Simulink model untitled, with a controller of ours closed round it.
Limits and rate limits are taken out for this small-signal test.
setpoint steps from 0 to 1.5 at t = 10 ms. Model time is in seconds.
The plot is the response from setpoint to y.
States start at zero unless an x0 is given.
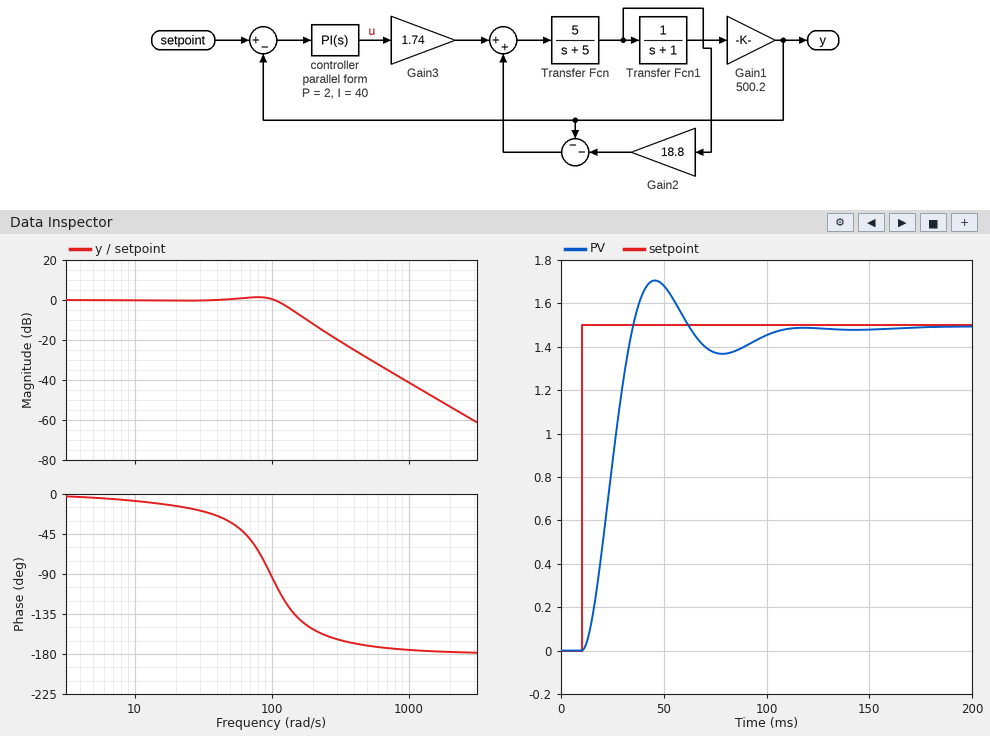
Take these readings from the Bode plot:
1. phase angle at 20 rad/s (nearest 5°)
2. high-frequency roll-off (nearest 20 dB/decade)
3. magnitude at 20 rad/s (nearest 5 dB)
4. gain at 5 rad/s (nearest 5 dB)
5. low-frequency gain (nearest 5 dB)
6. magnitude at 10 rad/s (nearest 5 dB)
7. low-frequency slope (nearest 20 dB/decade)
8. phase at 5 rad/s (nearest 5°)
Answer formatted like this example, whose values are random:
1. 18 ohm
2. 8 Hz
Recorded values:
1. -15°
2. -40 dB/decade
3. 0 dB
4. 0 dB
5. 0 dB
6. 0 dB
7. 0 dB/decade
8. -5°
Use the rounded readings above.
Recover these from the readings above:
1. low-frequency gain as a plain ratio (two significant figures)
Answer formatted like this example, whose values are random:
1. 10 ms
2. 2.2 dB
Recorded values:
1. 1.0
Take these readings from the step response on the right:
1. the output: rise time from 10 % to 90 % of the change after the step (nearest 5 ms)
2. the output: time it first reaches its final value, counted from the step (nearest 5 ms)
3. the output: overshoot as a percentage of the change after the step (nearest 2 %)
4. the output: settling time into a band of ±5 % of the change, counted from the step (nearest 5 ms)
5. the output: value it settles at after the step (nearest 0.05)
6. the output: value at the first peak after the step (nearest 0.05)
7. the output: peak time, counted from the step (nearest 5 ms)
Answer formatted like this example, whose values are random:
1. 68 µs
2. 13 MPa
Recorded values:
1. 15 ms
2. 25 ms
3. 14 %
4. 85 ms
5. 1.50
6. 1.70
7. 35 ms
